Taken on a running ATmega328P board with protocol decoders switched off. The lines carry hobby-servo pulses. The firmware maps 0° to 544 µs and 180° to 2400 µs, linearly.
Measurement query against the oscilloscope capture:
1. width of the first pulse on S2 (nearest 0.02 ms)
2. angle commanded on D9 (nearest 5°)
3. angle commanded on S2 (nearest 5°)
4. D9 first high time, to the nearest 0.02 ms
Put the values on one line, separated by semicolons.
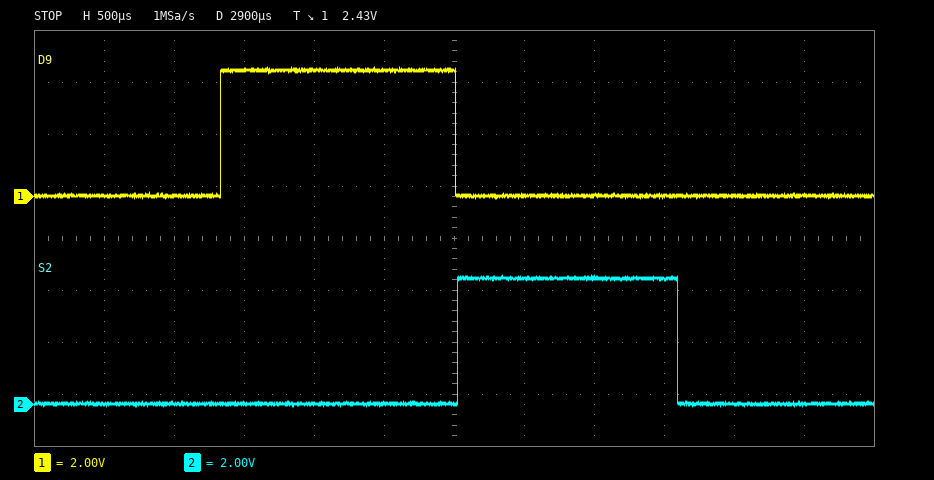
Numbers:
1.58 ms; 110°; 100°; 1.68 ms
